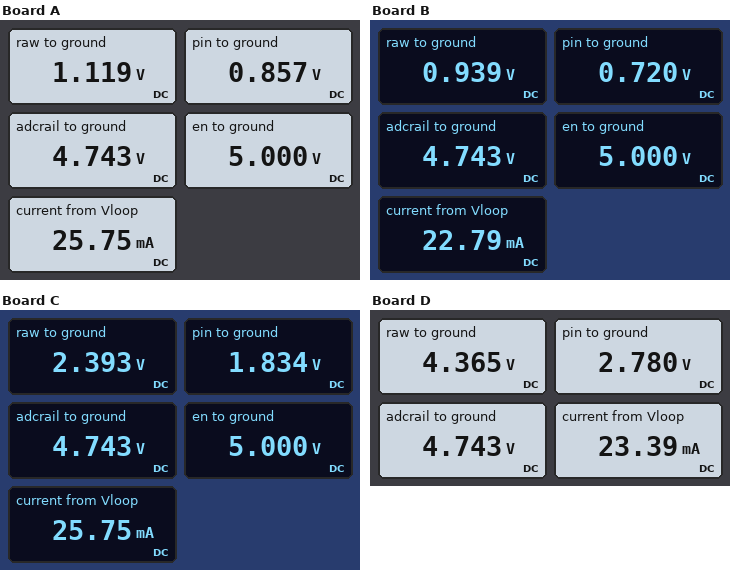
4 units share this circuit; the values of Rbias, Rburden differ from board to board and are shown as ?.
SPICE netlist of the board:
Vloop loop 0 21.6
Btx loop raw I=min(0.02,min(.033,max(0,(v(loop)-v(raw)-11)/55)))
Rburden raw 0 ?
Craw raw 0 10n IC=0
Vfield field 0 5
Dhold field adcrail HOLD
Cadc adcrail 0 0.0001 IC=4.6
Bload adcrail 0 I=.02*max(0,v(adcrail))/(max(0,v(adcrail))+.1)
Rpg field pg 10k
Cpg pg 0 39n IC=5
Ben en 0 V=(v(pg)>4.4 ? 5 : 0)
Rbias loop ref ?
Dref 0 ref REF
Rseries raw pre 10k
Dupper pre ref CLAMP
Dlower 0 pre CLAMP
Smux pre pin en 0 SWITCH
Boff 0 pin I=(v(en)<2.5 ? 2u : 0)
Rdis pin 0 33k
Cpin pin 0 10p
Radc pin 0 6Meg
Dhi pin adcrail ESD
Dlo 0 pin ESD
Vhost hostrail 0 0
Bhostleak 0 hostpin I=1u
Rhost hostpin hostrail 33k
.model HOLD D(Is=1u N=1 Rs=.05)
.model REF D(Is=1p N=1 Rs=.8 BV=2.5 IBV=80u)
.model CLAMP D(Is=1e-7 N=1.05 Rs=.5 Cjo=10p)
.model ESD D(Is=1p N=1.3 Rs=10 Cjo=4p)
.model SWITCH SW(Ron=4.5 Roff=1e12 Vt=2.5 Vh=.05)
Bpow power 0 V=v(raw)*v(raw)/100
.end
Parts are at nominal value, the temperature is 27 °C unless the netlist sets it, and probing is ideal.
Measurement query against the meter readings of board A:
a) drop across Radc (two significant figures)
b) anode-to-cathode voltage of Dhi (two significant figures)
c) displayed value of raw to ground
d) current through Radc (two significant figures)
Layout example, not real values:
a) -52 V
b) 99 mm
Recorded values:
a) 860 mV
b) -3.9 V
c) 1.119 V
d) 140 nA
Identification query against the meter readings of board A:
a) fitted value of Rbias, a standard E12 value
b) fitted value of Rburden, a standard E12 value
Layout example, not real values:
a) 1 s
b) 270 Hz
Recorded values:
a) 3.3 kΩ
b) 56 Ω
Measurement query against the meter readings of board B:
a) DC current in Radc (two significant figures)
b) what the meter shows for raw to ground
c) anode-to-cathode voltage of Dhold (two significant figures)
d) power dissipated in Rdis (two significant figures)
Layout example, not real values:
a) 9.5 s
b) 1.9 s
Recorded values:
a) 120 nA
b) 0.939 V
c) 260 mV
d) 16 µW
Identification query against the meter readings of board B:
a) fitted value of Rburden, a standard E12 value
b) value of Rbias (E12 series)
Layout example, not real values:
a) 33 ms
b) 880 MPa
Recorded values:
a) 47 Ω
b) 6.8 kΩ
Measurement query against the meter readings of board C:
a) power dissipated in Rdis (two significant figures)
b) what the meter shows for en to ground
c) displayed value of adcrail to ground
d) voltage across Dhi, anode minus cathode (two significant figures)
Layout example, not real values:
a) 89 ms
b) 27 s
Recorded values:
a) 100 µW
b) 5.000 V
c) 4.743 V
d) -2.9 V
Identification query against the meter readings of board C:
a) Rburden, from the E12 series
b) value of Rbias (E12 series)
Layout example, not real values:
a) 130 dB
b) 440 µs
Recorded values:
a) 120 Ω
b) 3.3 kΩ
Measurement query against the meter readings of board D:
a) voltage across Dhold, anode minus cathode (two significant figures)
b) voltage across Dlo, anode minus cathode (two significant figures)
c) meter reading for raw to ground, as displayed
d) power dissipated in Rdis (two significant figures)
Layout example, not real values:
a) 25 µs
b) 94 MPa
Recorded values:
a) 260 mV
b) -2.8 V
c) 4.365 V
d) 230 µW
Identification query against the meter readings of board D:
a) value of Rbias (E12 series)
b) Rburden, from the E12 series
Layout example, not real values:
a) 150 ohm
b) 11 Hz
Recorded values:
a) 5.6 kΩ
b) 220 Ω
